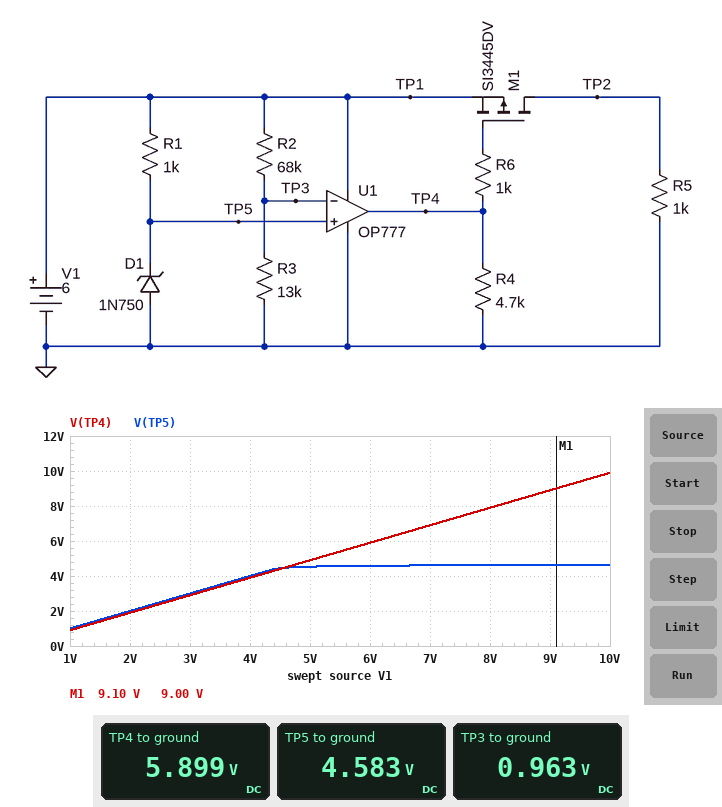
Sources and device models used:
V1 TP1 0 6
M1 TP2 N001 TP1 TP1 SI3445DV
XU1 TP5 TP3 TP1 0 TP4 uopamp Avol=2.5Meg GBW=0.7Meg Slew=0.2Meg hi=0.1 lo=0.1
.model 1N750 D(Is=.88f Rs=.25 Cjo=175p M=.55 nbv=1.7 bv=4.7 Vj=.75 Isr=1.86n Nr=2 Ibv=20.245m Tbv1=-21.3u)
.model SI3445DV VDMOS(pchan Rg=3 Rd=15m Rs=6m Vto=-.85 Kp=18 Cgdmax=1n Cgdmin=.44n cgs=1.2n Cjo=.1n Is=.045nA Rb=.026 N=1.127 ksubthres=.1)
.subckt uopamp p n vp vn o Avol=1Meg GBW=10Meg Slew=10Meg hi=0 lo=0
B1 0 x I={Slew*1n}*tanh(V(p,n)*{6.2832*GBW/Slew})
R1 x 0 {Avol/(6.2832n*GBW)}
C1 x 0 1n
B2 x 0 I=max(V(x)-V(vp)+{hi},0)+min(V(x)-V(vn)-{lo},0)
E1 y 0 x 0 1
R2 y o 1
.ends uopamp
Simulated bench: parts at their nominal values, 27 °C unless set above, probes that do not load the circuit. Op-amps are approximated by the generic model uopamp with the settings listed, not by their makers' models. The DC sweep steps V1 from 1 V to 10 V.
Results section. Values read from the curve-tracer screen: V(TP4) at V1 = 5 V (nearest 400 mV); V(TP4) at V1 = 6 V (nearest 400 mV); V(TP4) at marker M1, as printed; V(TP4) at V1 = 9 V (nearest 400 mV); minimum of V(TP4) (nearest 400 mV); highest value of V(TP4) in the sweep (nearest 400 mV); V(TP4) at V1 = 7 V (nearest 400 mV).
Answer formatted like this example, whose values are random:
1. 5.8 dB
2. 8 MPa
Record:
1. 4.8 V
2. 6.0 V
3. 9.00 V
4. 8.8 V
5. 800 mV
6. 10.0 V
7. 6.8 V
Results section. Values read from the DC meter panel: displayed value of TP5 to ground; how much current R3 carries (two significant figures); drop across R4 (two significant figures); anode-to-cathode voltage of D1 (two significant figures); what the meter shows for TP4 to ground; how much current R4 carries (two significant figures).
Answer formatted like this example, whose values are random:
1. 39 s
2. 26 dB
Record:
1. 4.583 V
2. 74 µA
3. 5.9 V
4. -4.6 V
5. 5.899 V
6. 1.3 mA
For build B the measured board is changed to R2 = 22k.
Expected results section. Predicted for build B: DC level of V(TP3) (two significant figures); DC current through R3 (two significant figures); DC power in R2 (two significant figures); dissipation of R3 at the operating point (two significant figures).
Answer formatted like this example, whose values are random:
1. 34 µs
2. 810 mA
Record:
1. 2.2 V
2. 170 µA
3. 650 µW
4. 380 µW
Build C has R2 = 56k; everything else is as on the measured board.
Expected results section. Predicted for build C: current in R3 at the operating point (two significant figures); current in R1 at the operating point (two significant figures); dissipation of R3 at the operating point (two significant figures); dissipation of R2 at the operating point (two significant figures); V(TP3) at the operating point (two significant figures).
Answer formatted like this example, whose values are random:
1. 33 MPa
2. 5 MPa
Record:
1. 87 µA
2. 1.4 mA
3. 98 µW
4. 420 µW
5. 1.1 V
